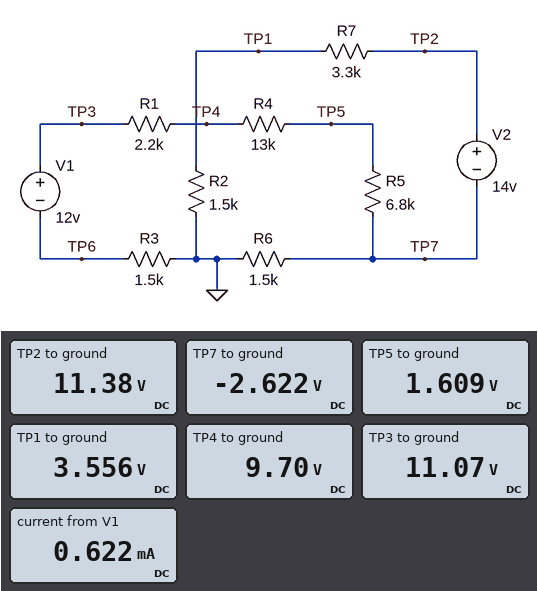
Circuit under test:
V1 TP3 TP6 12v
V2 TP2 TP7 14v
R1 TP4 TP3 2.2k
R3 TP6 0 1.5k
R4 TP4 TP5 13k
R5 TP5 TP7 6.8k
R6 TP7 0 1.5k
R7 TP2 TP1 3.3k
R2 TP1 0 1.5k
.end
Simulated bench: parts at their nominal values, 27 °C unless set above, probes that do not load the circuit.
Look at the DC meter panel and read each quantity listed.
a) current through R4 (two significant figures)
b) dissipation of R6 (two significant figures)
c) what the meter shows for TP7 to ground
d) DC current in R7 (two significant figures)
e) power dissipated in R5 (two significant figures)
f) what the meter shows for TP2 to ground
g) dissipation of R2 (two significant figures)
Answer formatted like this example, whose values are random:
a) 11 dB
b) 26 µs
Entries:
a) 620 µA
b) 4.6 mW
c) -2.622 V
d) 2.4 mA
e) 2.6 mW
f) 11.38 V
g) 8.4 mW
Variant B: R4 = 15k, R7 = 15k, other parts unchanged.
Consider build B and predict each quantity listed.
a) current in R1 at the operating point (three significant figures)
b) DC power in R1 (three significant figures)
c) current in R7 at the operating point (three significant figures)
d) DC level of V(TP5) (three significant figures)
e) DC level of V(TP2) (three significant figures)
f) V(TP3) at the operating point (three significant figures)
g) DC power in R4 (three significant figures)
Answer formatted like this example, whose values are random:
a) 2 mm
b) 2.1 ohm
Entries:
a) 490 µA
b) 528 µW
c) 819 µA
d) 2.84 V
e) 13.5 V
f) 11.3 V
g) 3.60 mW
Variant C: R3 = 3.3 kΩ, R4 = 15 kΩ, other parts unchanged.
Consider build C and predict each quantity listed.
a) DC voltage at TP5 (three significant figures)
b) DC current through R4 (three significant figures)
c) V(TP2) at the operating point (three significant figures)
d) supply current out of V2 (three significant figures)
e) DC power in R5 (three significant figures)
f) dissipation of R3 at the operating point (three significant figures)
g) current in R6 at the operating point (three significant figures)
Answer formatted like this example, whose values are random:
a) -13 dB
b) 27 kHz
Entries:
a) 949 mV
b) 539 µA
c) 11.3 V
d) 2.35 mA
e) 1.98 mW
f) 959 µW
g) 1.81 mA
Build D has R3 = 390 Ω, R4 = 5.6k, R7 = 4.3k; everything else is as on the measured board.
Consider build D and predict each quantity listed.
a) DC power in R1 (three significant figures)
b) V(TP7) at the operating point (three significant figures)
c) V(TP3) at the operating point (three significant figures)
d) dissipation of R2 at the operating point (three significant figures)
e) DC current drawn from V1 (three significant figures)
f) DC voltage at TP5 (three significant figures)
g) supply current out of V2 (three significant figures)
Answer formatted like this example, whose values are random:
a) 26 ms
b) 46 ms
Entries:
a) 1.86 mW
b) -1.78 V
c) 11.6 V
d) 6.66 mW
e) 919 µA
f) 4.47 V
g) 2.11 mA
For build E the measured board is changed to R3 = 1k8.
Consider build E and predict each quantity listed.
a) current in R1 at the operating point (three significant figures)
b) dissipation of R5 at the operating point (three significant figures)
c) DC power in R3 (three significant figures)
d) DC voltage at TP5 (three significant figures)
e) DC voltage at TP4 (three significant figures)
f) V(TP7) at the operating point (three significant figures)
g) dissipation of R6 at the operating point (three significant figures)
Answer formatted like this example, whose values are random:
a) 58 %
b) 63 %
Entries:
a) 615 µA
b) 2.57 mW
c) 680 µW
d) 1.55 V
e) 9.54 V
f) -2.63 V
g) 4.61 mW
